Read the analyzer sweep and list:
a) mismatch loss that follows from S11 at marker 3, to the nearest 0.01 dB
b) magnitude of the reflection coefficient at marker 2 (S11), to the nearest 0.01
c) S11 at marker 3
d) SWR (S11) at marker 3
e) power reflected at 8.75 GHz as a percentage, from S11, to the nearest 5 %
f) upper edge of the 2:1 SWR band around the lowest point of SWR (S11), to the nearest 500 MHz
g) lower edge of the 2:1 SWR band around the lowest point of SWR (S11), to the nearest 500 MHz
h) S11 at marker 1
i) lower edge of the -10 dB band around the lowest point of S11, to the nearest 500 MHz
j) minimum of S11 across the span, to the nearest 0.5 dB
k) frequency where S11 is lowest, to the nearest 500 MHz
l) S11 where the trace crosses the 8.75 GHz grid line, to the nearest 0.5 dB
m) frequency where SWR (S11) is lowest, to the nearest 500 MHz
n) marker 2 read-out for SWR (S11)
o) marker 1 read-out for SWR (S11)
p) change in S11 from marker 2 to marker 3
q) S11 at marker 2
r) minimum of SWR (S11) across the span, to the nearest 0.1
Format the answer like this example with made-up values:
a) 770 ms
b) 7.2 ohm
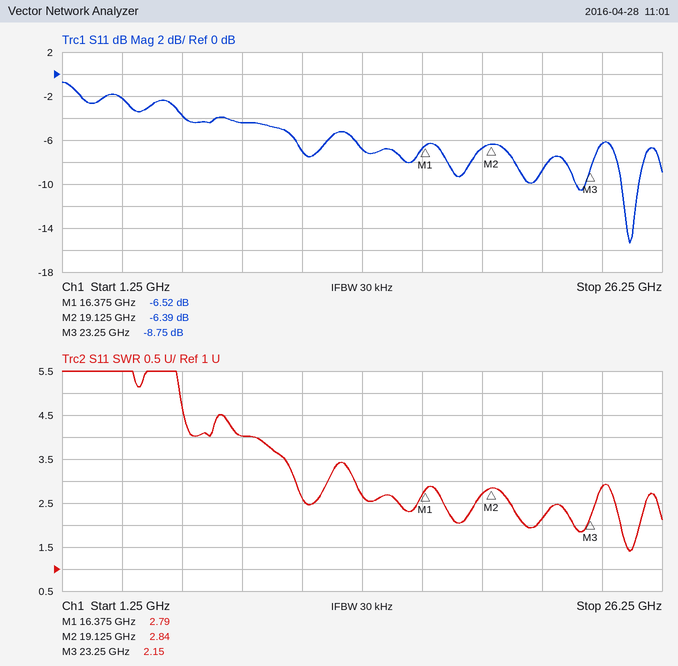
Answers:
a) 0.62 dB
b) 0.48
c) -8.75 dB
d) 2.15
e) 35 %
f) 25.5 GHz
g) 24.5 GHz
h) -6.52 dB
i) 24.5 GHz
j) -15.5 dB
k) 25.0 GHz
l) -4.5 dB
m) 25.0 GHz
n) 2.84
o) 2.79
p) -2.36 dB
q) -6.39 dB
r) 1.4
